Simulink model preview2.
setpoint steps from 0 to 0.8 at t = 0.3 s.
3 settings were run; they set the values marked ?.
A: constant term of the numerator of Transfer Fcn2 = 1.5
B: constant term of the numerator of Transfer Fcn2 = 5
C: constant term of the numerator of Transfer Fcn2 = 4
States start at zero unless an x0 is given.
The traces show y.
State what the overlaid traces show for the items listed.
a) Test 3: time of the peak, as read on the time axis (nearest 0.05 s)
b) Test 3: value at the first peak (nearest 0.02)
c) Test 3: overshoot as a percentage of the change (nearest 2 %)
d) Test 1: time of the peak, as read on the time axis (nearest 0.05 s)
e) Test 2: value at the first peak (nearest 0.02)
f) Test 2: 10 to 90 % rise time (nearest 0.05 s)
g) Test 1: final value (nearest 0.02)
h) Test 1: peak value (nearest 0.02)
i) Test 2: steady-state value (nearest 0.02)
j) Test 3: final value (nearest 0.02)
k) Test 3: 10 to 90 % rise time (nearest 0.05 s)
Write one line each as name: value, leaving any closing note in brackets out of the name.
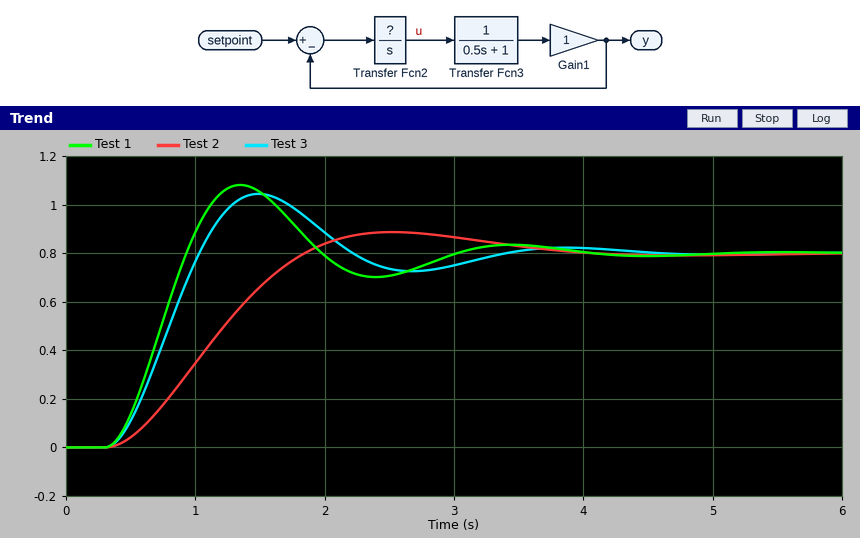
Test 3: time of the peak, as read on the time axis: 1.50 s
Test 3: value at the first peak: 1.04
Test 3: overshoot as a percentage of the change: 30 %
Test 1: time of the peak, as read on the time axis: 1.35 s
Test 2: value at the first peak: 0.88
Test 2: 10 to 90 % rise time: 1.05 s
Test 1: final value: 0.80
Test 1: peak value: 1.08
Test 2: steady-state value: 0.80
Test 3: final value: 0.80
Test 3: 10 to 90 % rise time: 0.50 s
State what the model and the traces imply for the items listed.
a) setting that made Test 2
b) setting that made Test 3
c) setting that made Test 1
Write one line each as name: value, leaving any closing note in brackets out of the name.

setting that made Test 2: A
setting that made Test 3: C
setting that made Test 1: B
